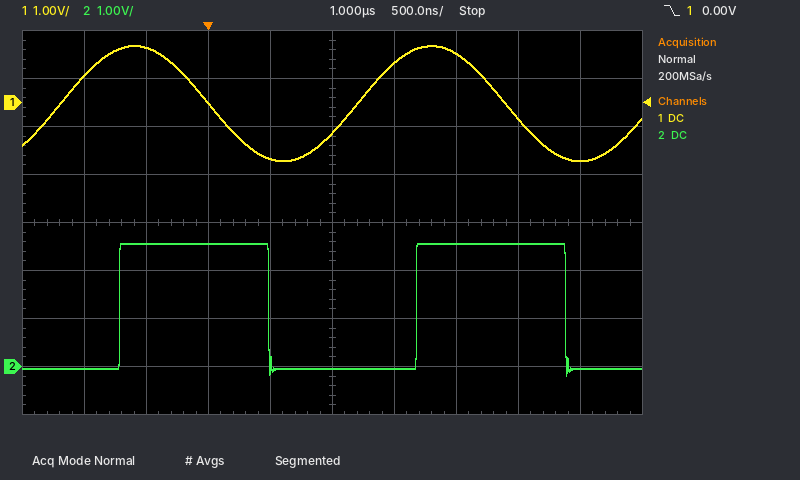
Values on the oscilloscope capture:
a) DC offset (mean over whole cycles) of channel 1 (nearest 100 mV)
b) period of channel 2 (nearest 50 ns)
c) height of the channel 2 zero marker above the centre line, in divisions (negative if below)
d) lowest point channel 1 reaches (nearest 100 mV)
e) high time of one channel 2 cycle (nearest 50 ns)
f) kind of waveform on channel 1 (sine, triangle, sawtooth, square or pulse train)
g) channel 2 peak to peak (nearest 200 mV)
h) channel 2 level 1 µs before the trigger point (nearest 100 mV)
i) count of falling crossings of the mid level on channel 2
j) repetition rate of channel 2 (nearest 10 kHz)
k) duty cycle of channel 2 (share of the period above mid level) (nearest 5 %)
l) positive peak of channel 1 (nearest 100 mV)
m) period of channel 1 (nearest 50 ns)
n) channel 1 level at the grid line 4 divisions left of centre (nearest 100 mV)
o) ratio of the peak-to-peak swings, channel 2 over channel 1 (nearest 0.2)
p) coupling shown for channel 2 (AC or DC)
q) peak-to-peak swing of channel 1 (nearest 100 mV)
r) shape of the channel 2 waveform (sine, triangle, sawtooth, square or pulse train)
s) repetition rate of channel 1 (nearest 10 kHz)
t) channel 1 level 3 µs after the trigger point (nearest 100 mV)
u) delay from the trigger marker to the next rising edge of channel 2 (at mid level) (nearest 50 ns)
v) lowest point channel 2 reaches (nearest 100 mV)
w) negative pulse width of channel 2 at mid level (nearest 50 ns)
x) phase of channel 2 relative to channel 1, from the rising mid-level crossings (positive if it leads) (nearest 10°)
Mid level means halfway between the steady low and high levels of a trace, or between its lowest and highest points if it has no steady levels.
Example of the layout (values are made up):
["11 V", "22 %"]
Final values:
["0.0 V", "2.40 µs", "-3.0 div", "-1.2 V", "1.20 µs", "sine", "2.8 V", "0.0 V", "2", "420 kHz", "50 %", "1.2 V", "2.40 µs", "600 mV", "1.2", "DC", "2.4 V", "square", "420 kHz", "-1.2 V", "1.70 µs", "-200 mV", "1.20 µs", "-70°"]
